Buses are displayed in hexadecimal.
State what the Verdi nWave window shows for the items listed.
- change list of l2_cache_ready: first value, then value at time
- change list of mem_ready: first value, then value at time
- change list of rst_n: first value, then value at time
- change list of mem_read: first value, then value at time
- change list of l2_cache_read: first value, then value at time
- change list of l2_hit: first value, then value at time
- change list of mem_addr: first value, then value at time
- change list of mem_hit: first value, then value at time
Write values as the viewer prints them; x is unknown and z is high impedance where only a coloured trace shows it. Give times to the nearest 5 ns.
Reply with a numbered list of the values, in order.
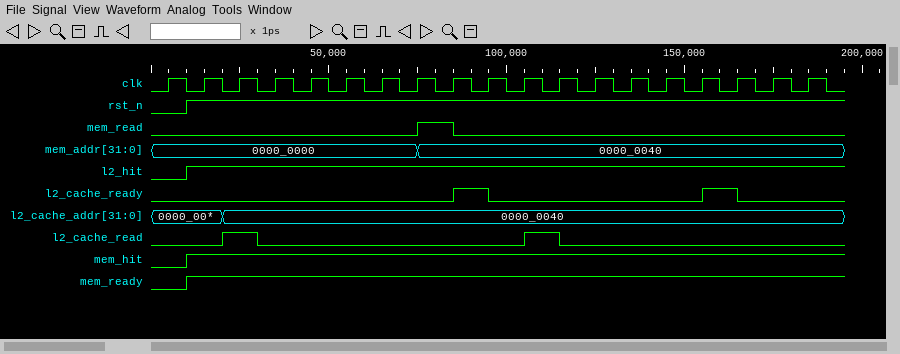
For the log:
1. 0, 1 at 85 ns, 0 at 95 ns, 1 at 155 ns, 0 at 165 ns
2. 0, 1 at 10 ns
3. 0, 1 at 10 ns
4. 0, 1 at 75 ns, 0 at 85 ns
5. 0, 1 at 20 ns, 0 at 30 ns, 1 at 105 ns, 0 at 115 ns
6. 0, 1 at 10 ns
7. 0000_0000, 0000_0040 at 75 ns
8. 0, 1 at 10 ns
